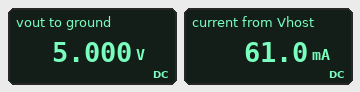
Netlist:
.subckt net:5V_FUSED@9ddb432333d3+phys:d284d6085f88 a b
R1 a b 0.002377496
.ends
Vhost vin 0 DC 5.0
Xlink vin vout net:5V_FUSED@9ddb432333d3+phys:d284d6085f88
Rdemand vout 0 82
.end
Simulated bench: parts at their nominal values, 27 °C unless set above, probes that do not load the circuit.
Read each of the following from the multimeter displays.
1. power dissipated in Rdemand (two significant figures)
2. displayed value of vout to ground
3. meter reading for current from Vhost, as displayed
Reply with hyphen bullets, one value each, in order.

- 300 mW
- 5.000 V
- 61.0 mA
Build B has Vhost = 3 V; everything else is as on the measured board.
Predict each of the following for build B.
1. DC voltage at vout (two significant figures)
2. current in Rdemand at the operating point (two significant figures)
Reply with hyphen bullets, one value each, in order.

- 3.0 V
- 37 mA
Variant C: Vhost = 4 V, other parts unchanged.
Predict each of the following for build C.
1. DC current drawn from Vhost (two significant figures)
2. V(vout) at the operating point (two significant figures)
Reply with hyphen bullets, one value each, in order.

- 49 mA
- 4.0 V
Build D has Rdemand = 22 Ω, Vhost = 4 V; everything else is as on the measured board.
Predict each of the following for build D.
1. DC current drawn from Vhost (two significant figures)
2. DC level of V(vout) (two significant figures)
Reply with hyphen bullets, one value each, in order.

- 180 mA
- 4.0 V
